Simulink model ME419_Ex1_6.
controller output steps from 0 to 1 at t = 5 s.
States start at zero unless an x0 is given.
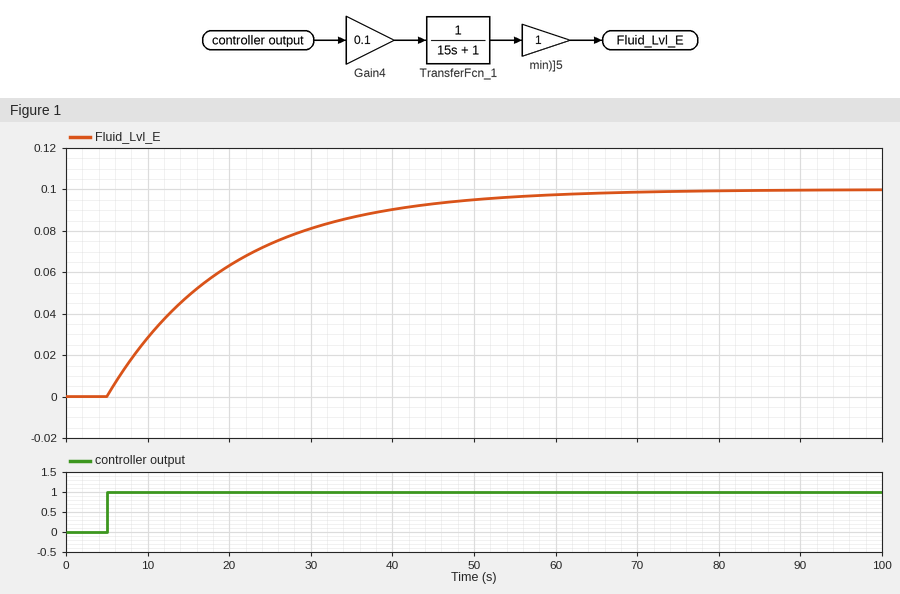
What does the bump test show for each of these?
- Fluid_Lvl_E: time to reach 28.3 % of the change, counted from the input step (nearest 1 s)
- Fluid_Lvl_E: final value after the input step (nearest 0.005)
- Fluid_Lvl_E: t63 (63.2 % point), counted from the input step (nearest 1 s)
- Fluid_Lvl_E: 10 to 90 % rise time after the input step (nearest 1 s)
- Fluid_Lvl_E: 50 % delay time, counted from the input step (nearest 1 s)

5 s
0.100
15 s
33 s
10 s
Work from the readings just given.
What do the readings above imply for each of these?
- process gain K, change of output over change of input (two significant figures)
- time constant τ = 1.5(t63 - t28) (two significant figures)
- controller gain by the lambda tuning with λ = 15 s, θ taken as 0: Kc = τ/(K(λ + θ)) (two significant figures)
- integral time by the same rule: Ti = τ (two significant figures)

0.10
15 s
10
15 s
